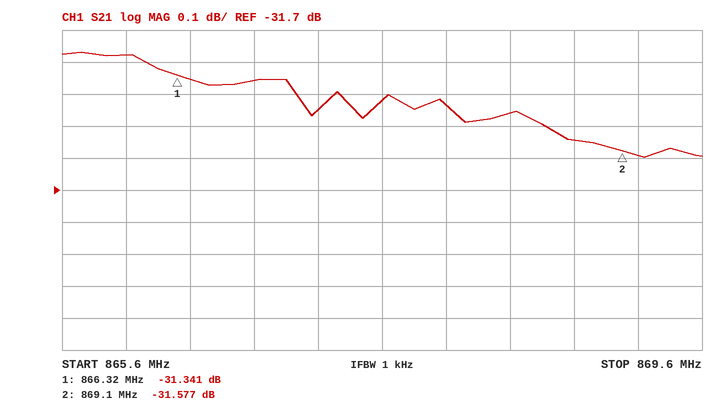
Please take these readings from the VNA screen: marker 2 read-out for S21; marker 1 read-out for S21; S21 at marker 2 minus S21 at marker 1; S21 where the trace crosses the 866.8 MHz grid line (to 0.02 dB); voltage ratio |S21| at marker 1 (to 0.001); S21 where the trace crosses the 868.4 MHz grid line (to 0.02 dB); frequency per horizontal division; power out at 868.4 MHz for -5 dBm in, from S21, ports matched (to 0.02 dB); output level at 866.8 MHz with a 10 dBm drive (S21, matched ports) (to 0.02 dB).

-31.577 dB
-31.341 dB
-0.236 dB
-31.36 dB
0.027
-31.46 dB
400 kHz
-36.46 dBm
-21.36 dBm
